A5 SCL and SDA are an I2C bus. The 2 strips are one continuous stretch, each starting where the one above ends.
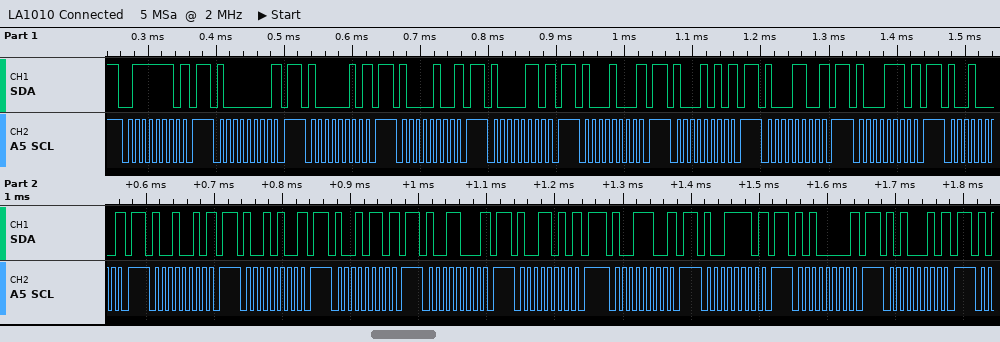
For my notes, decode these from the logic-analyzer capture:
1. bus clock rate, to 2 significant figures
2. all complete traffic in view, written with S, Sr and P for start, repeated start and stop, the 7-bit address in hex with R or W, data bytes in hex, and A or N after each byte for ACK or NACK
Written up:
100 kHz
S 3FW N P S 40W N P S 41W N P S 42W N P S 43W N P S 44W N P S 45W N P S 46W N P S 47W N P S 48W N P S 49W N P S 4AW N P S 4BW N P S 4CW N P S 4DW N P S 4EW N P S 4FW N P S 50W N P S 51W N P
